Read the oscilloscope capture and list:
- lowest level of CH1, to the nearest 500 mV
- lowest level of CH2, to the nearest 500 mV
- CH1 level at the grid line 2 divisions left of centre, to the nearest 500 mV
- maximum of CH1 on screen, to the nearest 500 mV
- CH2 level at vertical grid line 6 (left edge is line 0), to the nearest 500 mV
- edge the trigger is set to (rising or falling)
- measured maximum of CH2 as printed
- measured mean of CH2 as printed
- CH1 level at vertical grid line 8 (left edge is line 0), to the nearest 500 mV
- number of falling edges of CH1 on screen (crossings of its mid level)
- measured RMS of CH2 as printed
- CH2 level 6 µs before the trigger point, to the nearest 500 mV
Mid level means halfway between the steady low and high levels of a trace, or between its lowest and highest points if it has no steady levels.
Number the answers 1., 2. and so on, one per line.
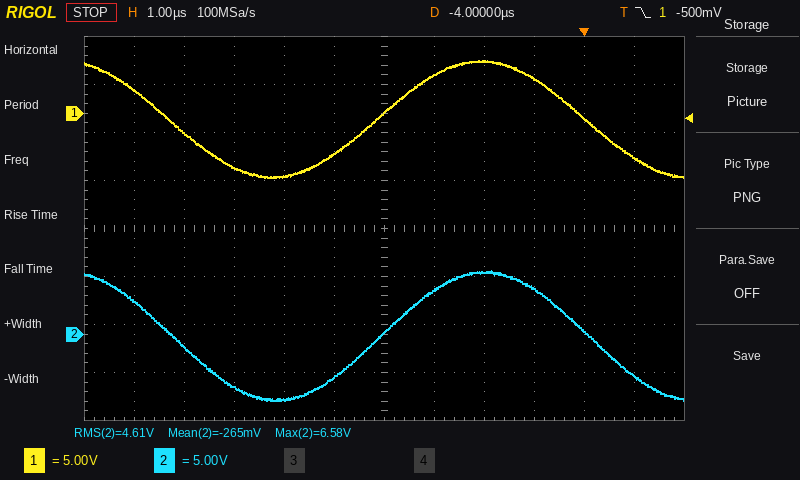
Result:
1. -6.5 V
2. -7.0 V
3. -6.5 V
4. 5.5 V
5. 0.0 V
6. falling
7. 6.58 V
8. -265 mV
9. 5.5 V
10. 2
11. 4.61 V
12. -7.0 V
